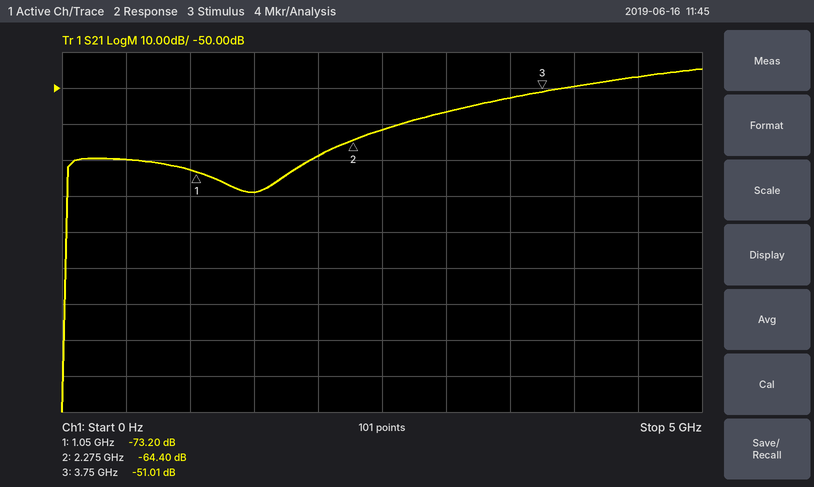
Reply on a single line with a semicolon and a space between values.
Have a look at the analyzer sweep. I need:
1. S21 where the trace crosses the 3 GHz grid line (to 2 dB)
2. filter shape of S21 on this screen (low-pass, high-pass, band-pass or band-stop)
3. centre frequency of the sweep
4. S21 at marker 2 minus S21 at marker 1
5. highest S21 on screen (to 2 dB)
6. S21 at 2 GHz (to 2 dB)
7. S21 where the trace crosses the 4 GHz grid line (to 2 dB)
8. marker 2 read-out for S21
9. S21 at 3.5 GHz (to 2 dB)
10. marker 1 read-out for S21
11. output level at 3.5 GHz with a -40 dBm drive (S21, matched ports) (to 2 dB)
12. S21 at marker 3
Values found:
-56 dB; high-pass; 2.5 GHz; 8.80 dB; -44 dB; -68 dB; -50 dB; -64.40 dB; -52 dB; -73.20 dB; -92 dBm; -51.01 dB
